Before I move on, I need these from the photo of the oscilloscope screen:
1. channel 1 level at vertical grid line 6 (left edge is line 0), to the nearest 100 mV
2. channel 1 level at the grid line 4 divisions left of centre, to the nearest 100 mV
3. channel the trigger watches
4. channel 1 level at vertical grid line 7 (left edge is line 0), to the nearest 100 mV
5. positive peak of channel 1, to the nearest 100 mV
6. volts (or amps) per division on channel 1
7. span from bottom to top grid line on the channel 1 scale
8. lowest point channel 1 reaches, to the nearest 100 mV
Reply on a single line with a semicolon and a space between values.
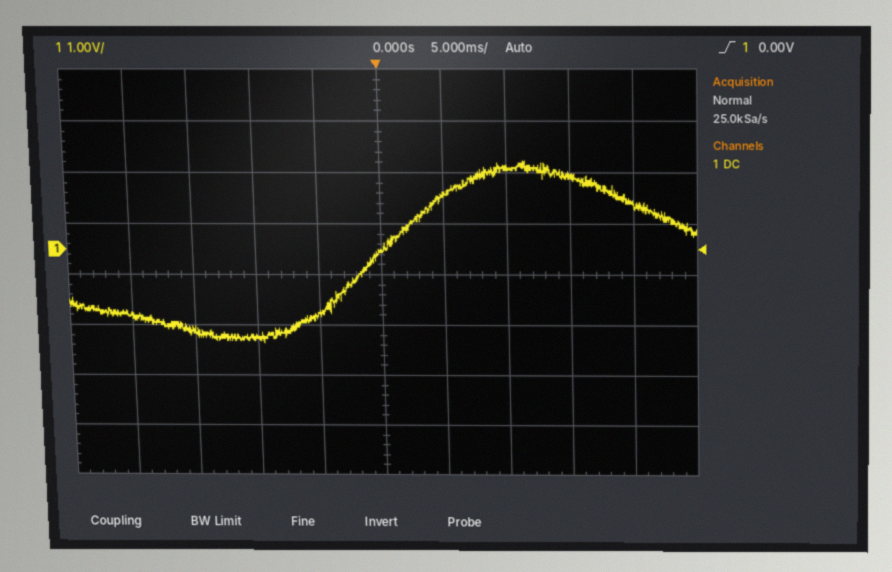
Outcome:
1.1 V; -1.3 V; channel 1; 1.6 V; 1.7 V; 1 V; 8 V; -1.8 V
